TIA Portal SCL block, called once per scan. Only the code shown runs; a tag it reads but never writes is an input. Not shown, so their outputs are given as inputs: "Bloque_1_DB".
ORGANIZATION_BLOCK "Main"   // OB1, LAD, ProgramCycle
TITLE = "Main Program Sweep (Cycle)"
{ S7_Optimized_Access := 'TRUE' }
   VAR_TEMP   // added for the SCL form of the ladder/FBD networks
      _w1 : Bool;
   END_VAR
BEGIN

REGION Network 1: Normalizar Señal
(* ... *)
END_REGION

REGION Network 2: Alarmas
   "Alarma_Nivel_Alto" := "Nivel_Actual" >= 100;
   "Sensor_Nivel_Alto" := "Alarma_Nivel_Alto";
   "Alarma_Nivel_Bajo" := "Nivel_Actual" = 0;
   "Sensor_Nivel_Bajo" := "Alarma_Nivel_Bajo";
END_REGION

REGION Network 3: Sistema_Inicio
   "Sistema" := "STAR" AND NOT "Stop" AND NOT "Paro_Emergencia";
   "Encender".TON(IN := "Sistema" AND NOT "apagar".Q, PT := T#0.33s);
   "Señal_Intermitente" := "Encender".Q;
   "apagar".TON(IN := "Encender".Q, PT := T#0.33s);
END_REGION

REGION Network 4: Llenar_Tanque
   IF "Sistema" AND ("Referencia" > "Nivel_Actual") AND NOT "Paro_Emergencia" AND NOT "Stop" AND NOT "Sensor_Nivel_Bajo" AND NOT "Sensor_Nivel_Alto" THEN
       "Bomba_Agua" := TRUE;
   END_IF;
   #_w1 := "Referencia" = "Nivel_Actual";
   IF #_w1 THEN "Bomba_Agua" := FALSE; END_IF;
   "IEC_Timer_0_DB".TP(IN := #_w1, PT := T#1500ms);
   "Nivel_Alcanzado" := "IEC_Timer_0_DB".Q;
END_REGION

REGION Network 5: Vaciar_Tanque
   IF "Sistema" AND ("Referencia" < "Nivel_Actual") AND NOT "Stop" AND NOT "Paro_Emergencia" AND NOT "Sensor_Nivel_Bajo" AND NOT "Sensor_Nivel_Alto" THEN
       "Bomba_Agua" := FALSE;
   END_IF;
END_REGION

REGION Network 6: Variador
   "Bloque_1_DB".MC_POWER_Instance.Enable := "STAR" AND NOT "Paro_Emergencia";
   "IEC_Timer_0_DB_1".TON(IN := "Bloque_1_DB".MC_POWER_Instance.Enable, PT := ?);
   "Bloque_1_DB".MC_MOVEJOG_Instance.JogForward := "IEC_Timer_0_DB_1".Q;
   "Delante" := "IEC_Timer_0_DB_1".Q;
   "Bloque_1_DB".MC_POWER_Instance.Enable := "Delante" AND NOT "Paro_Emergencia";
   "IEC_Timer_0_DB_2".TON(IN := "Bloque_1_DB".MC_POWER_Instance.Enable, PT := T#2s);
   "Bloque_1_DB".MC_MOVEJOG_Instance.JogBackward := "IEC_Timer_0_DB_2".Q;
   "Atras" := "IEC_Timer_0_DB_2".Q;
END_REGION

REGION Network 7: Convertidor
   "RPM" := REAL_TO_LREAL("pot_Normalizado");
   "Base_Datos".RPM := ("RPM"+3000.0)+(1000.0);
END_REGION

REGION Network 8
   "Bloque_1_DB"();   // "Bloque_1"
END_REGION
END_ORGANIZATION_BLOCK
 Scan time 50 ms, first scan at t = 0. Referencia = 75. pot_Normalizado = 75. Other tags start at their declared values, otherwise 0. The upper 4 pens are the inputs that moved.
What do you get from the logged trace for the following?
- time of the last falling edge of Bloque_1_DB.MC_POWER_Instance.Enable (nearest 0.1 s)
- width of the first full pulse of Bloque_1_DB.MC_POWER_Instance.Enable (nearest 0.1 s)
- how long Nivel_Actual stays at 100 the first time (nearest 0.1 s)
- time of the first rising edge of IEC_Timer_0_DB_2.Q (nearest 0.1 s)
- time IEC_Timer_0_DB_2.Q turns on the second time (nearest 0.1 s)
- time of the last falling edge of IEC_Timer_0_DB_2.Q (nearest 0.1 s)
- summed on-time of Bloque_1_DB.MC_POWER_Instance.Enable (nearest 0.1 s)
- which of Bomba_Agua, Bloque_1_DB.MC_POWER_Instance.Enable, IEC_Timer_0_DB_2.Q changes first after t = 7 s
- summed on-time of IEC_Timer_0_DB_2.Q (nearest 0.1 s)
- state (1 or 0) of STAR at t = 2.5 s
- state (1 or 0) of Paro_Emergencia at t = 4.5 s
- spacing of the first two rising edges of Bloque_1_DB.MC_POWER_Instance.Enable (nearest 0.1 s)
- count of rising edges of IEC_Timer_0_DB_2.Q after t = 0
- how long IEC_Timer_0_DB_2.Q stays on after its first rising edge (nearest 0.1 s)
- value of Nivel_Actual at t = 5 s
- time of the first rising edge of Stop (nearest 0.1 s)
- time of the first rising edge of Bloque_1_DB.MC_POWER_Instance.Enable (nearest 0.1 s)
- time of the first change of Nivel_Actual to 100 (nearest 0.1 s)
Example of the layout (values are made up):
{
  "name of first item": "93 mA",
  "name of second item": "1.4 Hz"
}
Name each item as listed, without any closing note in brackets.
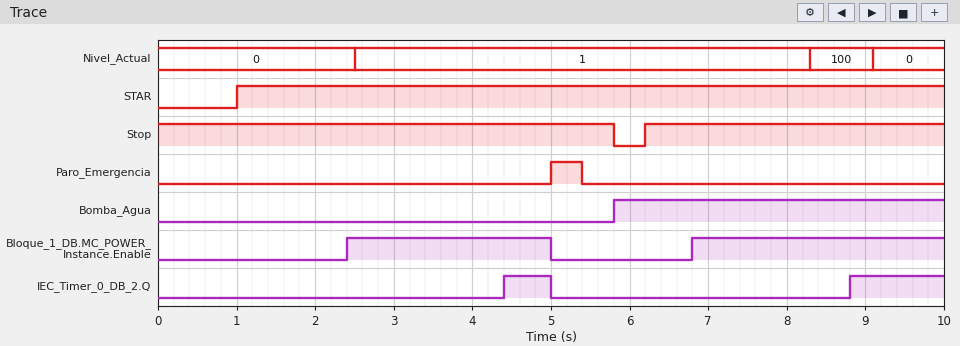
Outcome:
{
  "time of the last falling edge of Bloque_1_DB.MC_POWER_Instance.Enable": "5.0 s",
  "width of the first full pulse of Bloque_1_DB.MC_POWER_Instance.Enable": "2.6 s",
  "how long Nivel_Actual stays at 100 the first time": "0.8 s",
  "time of the first rising edge of IEC_Timer_0_DB_2.Q": "4.4 s",
  "time IEC_Timer_0_DB_2.Q turns on the second time": "8.8 s",
  "time of the last falling edge of IEC_Timer_0_DB_2.Q": "5.0 s",
  "summed on-time of Bloque_1_DB.MC_POWER_Instance.Enable": "5.8 s",
  "which of Bomba_Agua, Bloque_1_DB.MC_POWER_Instance.Enable, IEC_Timer_0_DB_2.Q changes first after t = 7 s": "IEC_Timer_0_DB_2.Q",
  "summed on-time of IEC_Timer_0_DB_2.Q": "1.8 s",
  "state (1 or 0) of STAR at t = 2.5 s": "1",
  "state (1 or 0) of Paro_Emergencia at t = 4.5 s": "0",
  "spacing of the first two rising edges of Bloque_1_DB.MC_POWER_Instance.Enable": "4.4 s",
  "count of rising edges of IEC_Timer_0_DB_2.Q after t = 0": "2",
  "how long IEC_Timer_0_DB_2.Q stays on after its first rising edge": "0.6 s",
  "value of Nivel_Actual at t = 5 s": "1",
  "time of the first rising edge of Stop": "6.2 s",
  "time of the first rising edge of Bloque_1_DB.MC_POWER_Instance.Enable": "2.4 s",
  "time of the first change of Nivel_Actual to 100": "8.3 s"
}
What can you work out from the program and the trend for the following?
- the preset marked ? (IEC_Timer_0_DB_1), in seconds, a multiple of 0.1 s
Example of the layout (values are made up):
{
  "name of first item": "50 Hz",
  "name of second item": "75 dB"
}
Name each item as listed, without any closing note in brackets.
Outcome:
{
  "the preset marked ? (IEC_Timer_0_DB_1), in seconds, a multiple of 0.1 s": "1.4 s"
}
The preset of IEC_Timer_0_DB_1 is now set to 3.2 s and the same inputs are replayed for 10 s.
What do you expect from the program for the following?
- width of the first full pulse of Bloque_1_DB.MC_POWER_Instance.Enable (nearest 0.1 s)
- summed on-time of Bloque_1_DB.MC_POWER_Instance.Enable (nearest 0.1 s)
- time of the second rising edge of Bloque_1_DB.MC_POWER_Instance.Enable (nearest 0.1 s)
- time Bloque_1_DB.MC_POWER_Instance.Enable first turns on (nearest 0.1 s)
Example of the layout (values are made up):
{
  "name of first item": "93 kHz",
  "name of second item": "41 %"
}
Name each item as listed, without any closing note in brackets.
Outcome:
{
  "width of the first full pulse of Bloque_1_DB.MC_POWER_Instance.Enable": "0.8 s",
  "summed on-time of Bloque_1_DB.MC_POWER_Instance.Enable": "2.2 s",
  "time of the second rising edge of Bloque_1_DB.MC_POWER_Instance.Enable": "8.6 s",
  "time Bloque_1_DB.MC_POWER_Instance.Enable first turns on": "4.2 s"
}
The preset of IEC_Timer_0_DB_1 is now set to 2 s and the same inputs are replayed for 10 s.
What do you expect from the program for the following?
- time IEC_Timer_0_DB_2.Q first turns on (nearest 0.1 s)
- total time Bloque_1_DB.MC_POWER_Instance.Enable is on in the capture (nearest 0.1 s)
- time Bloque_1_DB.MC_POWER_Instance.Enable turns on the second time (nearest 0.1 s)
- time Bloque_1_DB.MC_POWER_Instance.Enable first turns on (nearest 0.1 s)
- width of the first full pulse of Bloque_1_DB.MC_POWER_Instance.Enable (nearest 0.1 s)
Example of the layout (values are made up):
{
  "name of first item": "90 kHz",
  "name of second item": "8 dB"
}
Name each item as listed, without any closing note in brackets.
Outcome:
{
  "time IEC_Timer_0_DB_2.Q first turns on": "9.4 s",
  "total time Bloque_1_DB.MC_POWER_Instance.Enable is on in the capture": "4.6 s",
  "time Bloque_1_DB.MC_POWER_Instance.Enable turns on the second time": "7.4 s",
  "time Bloque_1_DB.MC_POWER_Instance.Enable first turns on": "3.0 s",
  "width of the first full pulse of Bloque_1_DB.MC_POWER_Instance.Enable": "2.0 s"
}
